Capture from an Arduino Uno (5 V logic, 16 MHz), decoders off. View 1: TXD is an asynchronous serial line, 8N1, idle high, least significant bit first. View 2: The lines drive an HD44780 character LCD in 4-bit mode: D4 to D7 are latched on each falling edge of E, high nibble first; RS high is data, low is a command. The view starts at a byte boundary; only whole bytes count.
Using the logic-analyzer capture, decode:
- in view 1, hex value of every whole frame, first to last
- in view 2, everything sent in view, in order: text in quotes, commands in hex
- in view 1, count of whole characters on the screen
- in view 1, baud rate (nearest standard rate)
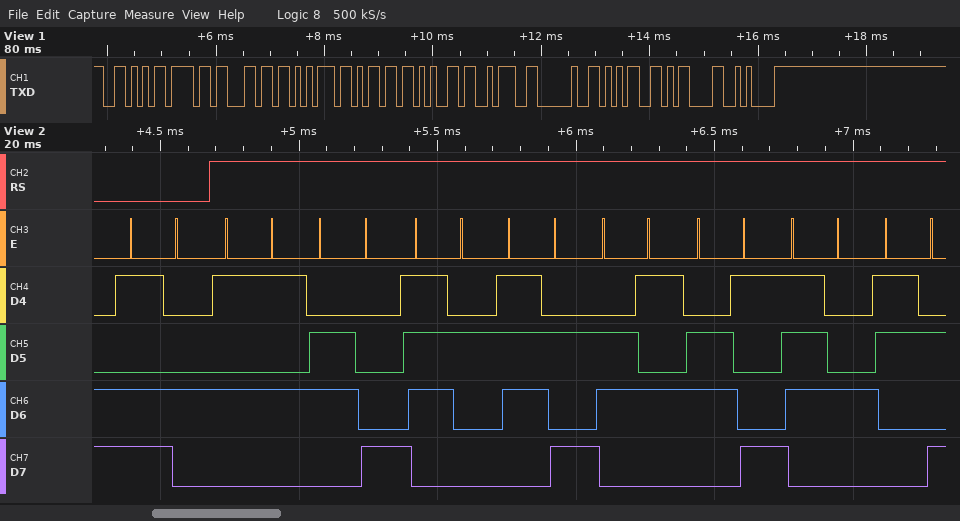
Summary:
0x56 0x6F 0x6C 0x75 0x6D 0x65 0x3A 0x20 0x35 0x0D 0x0A
0xD4 "Uhrzeit:"
11
9600 baud
